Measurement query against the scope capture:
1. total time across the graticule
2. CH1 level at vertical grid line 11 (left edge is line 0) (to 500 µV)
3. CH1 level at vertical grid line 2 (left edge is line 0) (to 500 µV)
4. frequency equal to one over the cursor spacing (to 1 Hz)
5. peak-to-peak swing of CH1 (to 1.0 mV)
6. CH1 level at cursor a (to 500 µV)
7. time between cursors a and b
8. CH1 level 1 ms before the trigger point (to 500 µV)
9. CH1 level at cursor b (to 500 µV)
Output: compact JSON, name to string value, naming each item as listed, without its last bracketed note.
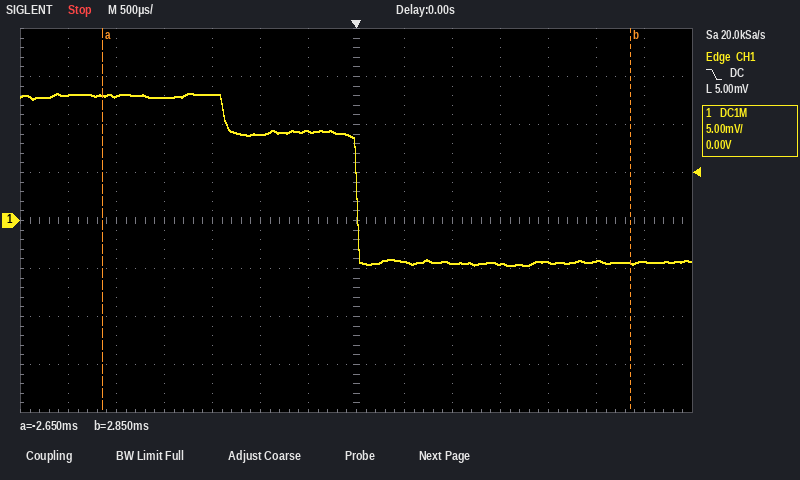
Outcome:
{"total time across the graticule": "7 ms", "CH1 level at vertical grid line 11 (left edge is line 0)": "-4.5 mV", "CH1 level at vertical grid line 2 (left edge is line 0)": "13.0 mV", "frequency equal to one over the cursor spacing": "182 Hz", "peak-to-peak swing of CH1": "18.0 mV", "CH1 level at cursor a": "13.0 mV", "time between cursors a and b": "5.50 ms", "CH1 level 1 ms before the trigger point": "9.0 mV", "CH1 level at cursor b": "-4.5 mV"}
